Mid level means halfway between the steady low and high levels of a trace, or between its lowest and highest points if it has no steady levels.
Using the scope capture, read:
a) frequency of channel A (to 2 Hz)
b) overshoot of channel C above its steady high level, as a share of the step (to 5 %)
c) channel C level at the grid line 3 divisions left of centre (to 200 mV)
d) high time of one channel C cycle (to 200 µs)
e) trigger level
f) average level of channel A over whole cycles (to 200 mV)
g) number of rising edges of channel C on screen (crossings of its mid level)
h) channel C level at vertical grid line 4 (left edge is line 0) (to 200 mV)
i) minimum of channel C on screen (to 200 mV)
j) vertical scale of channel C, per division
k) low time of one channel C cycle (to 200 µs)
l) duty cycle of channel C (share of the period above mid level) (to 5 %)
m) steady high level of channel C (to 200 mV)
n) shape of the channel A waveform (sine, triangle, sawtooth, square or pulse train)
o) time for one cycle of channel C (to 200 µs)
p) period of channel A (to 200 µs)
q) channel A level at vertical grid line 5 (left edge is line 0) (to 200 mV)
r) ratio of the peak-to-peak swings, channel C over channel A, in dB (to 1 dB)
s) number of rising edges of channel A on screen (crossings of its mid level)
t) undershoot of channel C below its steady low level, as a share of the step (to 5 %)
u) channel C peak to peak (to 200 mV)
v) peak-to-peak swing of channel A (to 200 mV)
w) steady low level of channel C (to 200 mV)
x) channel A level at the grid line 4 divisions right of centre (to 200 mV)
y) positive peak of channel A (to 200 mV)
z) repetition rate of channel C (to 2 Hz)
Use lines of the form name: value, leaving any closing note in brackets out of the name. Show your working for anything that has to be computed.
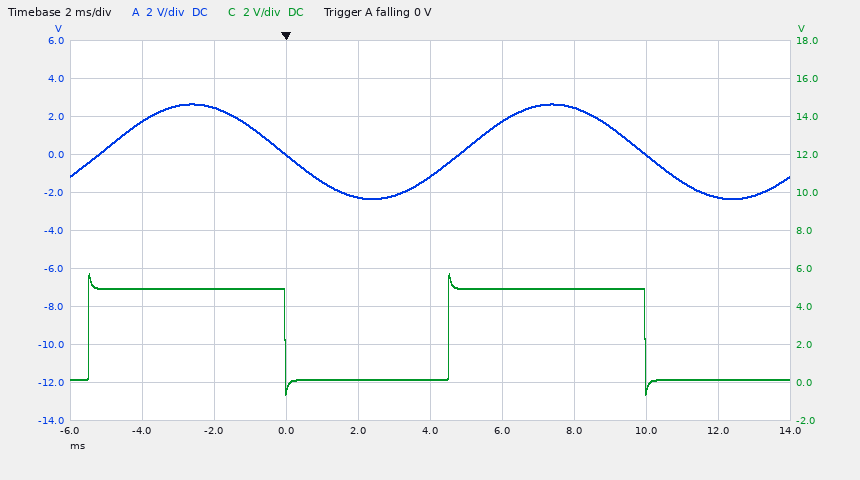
frequency of channel A: 1 / 10.0 ms ≈ 100 Hz
overshoot of channel C above its steady high level, as a share of the step: 15 %
channel C level at the grid line 3 divisions left of centre: 5.0 V
high time of one channel C cycle: 5.4 ms
trigger level: 0 V
average level of channel A over whole cycles: (2.6 V + (-2.4 V)) / 2 ≈ 100 mV, so 200 mV to the nearest 200 mV
number of rising edges of channel C on screen: 2
channel C level at vertical grid line 4 (left edge is line 0): 200 mV
minimum of channel C on screen: -600 mV
vertical scale of channel C, per division: 2 V
low time of one channel C cycle: 4.6 ms
duty cycle of channel C (share of the period above mid level): 5.4 ms / 10.0 ms ≈ 54.0 %, so 55 % to the nearest 5 %
steady high level of channel C: 5.0 V
shape of the channel A waveform: sine
time for one cycle of channel C: 10.0 ms
period of channel A: 10.0 ms
channel A level at vertical grid line 5 (left edge is line 0): -1.2 V
ratio of the peak-to-peak swings, channel C over channel A, in dB: 20 log10(6.4 V / 5.0 V) ≈ 2 dB
number of rising edges of channel A on screen: 2
undershoot of channel C below its steady low level, as a share of the step: 15 %
channel C peak to peak: 5.8 V − (-600 mV) = 6.4 V
peak-to-peak swing of channel A: 2.6 V − (-2.4 V) = 5.0 V
steady low level of channel C: 200 mV
channel A level at the grid line 4 divisions right of centre: -2.2 V
positive peak of channel A: 2.6 V
repetition rate of channel C: 1 / 10.0 ms ≈ 100 Hz
